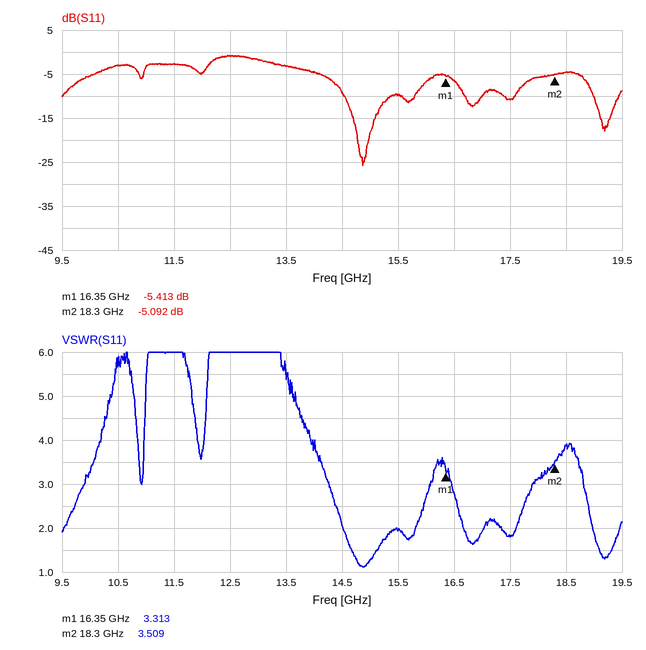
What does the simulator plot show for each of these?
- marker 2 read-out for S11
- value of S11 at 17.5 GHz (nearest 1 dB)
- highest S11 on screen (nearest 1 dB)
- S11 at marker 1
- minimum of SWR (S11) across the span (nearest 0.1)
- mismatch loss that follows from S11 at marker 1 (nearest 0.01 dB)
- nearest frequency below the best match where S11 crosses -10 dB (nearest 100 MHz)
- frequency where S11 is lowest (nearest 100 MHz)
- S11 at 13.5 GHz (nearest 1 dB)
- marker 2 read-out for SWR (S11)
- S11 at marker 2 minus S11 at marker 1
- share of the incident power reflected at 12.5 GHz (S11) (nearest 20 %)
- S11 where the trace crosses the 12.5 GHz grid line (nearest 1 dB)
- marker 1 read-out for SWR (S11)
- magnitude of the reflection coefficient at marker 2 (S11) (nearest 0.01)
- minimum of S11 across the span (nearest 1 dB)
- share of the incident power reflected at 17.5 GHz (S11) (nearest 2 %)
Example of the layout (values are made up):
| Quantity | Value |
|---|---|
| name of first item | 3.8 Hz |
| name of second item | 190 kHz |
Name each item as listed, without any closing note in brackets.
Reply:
| Quantity | Value |
|---|---|
| marker 2 read-out for S11 | -5.092 dB |
| value of S11 at 17.5 GHz | -11 dB |
| highest S11 on screen | -1 dB |
| S11 at marker 1 | -5.413 dB |
| minimum of SWR (S11) across the span | 1.1 |
| mismatch loss that follows from S11 at marker 1 | 1.47 dB |
| nearest frequency below the best match where S11 crosses -10 dB | 14.5 GHz |
| frequency where S11 is lowest | 14.9 GHz |
| S11 at 13.5 GHz | -3 dB |
| marker 2 read-out for SWR | 3.509 |
| S11 at marker 2 minus S11 at marker 1 | 0.321 dB |
| share of the incident power reflected at 12.5 GHz (S11) | 80 % |
| S11 where the trace crosses the 12.5 GHz grid line | -1 dB |
| marker 1 read-out for SWR | 3.313 |
| magnitude of the reflection coefficient at marker 2 (S11) | 0.56 |
| minimum of S11 across the span | -26 dB |
| share of the incident power reflected at 17.5 GHz (S11) | 8 % |
